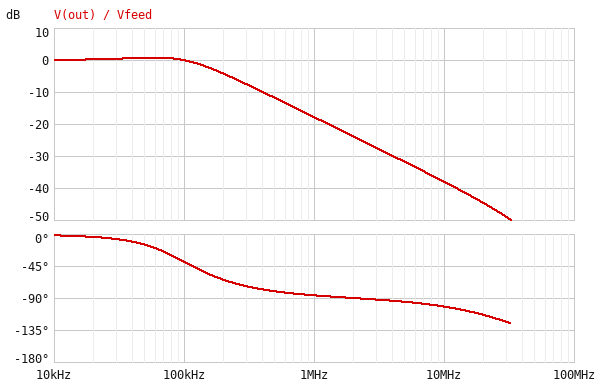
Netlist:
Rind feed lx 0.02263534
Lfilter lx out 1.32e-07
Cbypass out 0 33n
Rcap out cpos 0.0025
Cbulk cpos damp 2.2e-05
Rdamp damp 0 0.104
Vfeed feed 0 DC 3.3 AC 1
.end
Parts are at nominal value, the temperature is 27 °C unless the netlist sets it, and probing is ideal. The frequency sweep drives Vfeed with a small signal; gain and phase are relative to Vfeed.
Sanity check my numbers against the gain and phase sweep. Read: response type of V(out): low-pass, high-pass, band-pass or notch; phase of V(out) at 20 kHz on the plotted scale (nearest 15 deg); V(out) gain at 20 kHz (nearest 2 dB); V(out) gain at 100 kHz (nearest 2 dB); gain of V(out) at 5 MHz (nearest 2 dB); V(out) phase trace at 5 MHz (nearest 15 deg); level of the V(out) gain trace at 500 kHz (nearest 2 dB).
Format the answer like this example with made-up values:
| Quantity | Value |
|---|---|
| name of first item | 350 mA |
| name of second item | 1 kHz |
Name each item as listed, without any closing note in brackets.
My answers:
| Quantity | Value |
|---|---|
| response type of V(out): low-pass, high-pass, band-pass or notch | low-pass |
| phase of V(out) at 20 kHz on the plotted scale | 0 deg |
| V(out) gain at 20 kHz | 0 dB |
| V(out) gain at 100 kHz | 0 dB |
| gain of V(out) at 5 MHz | -32 dB |
| V(out) phase trace at 5 MHz | -90 deg |
| level of the V(out) gain trace at 500 kHz | -12 dB |
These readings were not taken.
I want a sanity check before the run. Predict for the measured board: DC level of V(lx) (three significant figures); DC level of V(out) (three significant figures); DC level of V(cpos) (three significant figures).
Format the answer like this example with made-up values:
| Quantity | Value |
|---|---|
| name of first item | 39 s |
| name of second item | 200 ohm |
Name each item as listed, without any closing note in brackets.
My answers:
| Quantity | Value |
|---|---|
| DC level of V(lx) | 3.30 V |
| DC level of V(out) | 3.30 V |
| DC level of V(cpos) | 3.30 V |
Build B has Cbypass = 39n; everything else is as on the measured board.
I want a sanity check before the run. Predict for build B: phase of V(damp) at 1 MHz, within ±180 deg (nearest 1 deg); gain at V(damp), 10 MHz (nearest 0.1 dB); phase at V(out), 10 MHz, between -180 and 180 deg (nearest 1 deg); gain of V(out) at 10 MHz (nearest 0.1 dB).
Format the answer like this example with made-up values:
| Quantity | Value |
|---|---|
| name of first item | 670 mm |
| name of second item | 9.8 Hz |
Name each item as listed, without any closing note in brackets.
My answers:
| Quantity | Value |
|---|---|
| phase of V(damp) at 1 MHz, within ±180 deg | -83 deg |
| gain at V(damp), 10 MHz | -38.3 dB |
| phase at V(out), 10 MHz, between -180 and 180 deg | -104 deg |
| gain of V(out) at 10 MHz | -38.1 dB |
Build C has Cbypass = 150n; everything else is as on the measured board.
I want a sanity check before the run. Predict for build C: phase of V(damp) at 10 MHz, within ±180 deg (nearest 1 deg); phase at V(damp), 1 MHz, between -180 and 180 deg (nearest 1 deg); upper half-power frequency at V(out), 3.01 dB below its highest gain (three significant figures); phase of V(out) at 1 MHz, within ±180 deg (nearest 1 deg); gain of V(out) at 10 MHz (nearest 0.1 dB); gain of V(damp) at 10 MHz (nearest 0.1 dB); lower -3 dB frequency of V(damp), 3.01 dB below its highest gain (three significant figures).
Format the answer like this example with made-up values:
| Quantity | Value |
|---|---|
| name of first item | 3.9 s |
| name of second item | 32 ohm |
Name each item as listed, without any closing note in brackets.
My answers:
| Quantity | Value |
|---|---|
| phase of V(damp) at 10 MHz, within ±180 deg | -134 deg |
| phase at V(damp), 1 MHz, between -180 and 180 deg | -87 deg |
| upper half-power frequency at V(out), 3.01 dB below its highest gain | 153 kHz |
| phase of V(out) at 1 MHz, within ±180 deg | -91 deg |
| gain of V(out) at 10 MHz | -40.8 dB |
| gain of V(damp) at 10 MHz | -41.0 dB |
| lower -3 dB frequency of V(damp), 3.01 dB below its highest gain | 43.9 kHz |
